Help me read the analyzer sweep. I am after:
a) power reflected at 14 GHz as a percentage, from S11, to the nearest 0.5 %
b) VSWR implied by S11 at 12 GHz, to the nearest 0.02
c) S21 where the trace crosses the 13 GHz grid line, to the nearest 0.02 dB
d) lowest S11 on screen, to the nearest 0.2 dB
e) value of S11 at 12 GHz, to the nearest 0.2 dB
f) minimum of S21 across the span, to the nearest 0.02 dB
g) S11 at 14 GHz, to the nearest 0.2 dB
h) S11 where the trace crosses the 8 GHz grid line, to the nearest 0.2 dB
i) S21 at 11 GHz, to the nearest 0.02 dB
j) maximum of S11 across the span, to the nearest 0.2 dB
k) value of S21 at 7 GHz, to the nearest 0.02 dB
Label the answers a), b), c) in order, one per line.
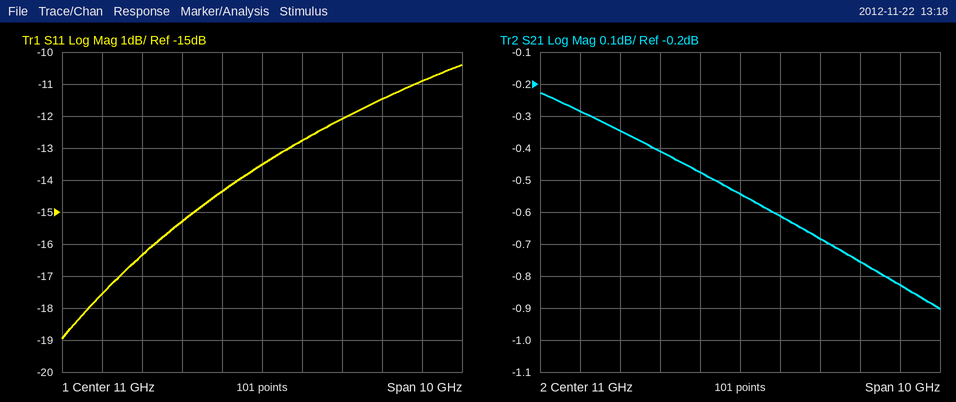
a) 7.0 %
b) 1.60
c) -0.68 dB
d) -19.0 dB
e) -12.8 dB
f) -0.90 dB
g) -11.4 dB
h) -16.4 dB
i) -0.54 dB
j) -10.4 dB
k) -0.28 dB
